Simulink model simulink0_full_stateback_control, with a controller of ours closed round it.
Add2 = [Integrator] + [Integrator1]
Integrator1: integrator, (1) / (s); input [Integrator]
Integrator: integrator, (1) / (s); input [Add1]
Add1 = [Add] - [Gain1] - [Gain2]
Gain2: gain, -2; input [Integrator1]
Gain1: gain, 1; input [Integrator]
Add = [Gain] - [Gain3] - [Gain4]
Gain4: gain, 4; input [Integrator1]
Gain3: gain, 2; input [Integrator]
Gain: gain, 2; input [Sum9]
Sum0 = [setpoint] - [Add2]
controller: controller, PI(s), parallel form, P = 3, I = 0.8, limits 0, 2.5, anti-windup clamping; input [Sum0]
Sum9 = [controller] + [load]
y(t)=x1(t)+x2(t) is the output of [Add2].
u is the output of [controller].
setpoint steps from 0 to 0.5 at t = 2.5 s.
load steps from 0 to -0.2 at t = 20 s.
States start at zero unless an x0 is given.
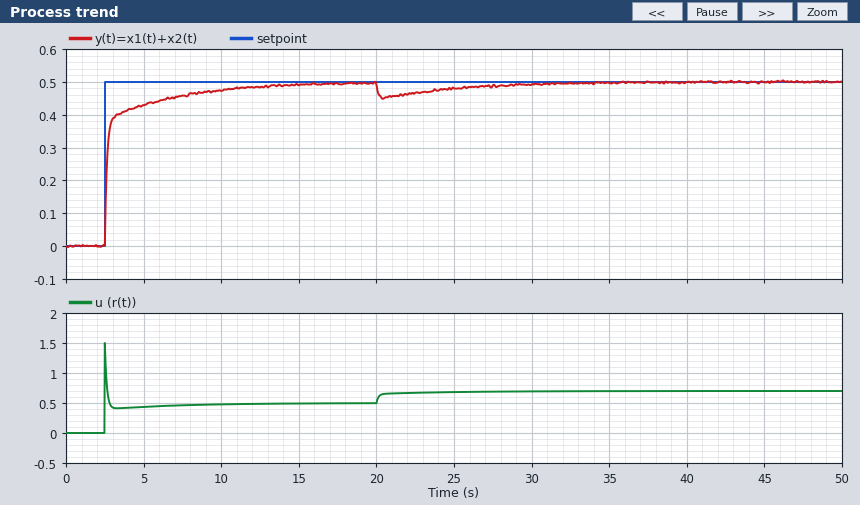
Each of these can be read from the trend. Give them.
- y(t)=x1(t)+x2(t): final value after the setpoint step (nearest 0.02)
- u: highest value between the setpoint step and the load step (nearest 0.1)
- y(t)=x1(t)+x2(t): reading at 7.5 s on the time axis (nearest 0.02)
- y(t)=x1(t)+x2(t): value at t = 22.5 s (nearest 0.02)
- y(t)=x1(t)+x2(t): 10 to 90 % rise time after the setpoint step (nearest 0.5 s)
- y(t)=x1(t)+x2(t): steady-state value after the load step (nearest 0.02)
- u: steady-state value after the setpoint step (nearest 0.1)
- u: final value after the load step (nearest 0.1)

0.50
1.5
0.46
0.46
4.0 s
0.50
0.5
0.7
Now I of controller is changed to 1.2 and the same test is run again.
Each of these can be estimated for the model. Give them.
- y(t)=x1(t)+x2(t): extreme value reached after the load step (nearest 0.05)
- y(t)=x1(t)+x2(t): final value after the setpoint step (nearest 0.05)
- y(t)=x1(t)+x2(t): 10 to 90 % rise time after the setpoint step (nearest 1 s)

0.45
0.50
3 s
